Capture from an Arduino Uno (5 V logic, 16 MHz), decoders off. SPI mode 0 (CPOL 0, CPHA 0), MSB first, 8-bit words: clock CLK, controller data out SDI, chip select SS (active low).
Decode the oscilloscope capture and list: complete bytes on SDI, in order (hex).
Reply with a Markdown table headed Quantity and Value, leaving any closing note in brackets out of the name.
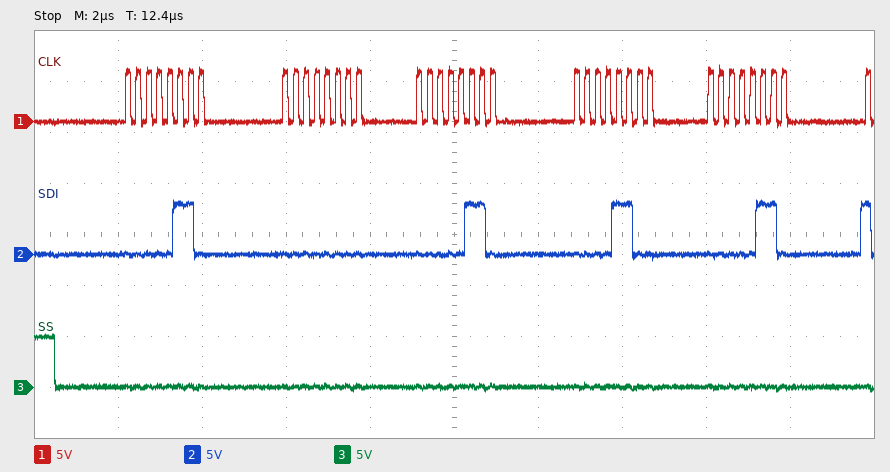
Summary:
| Quantity | Value |
|---|---|
| complete bytes on SDI, in order | 0x06 0x00 0x06 0x0C 0x06 |
